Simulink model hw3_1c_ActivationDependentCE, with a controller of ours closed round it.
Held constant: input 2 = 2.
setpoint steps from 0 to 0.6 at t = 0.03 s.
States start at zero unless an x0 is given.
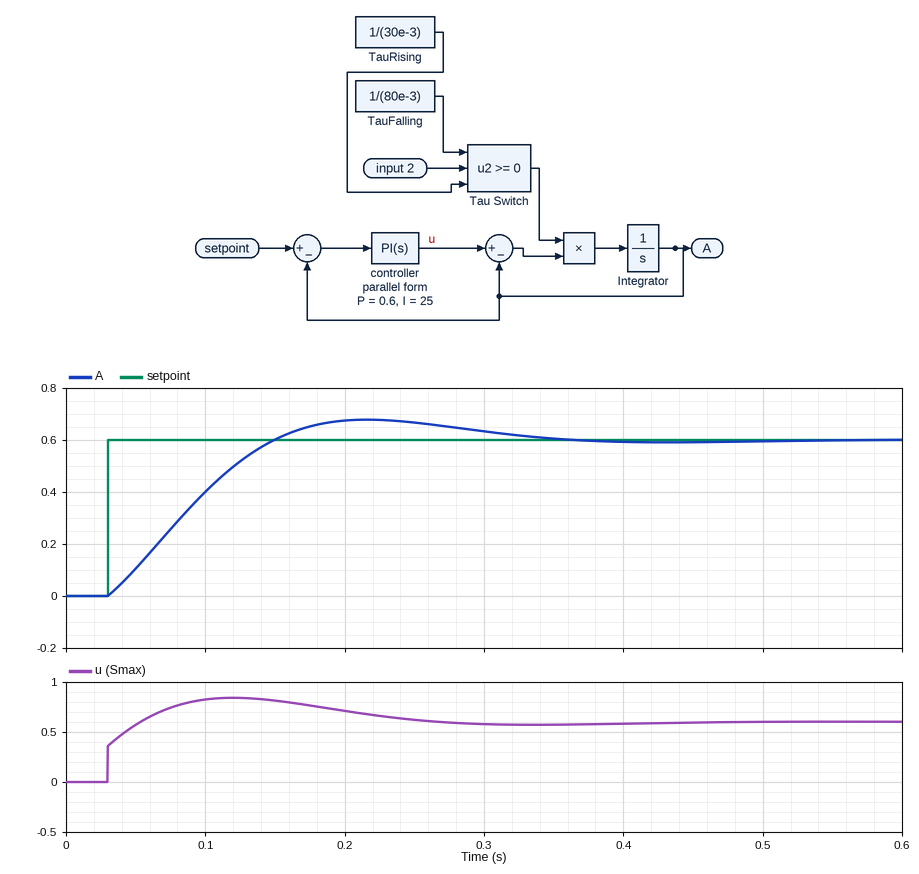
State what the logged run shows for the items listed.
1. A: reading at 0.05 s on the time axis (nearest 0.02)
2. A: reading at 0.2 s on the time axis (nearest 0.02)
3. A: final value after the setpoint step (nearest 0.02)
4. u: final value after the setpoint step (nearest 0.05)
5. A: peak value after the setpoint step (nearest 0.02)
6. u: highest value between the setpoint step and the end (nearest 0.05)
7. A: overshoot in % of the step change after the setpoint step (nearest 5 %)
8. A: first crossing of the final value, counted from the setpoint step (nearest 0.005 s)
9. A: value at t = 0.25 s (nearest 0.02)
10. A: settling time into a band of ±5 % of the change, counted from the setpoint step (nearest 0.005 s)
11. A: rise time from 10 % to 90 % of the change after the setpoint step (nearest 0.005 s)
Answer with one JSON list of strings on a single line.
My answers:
["0.10", "0.68", "0.60", "0.60", "0.68", "0.85", "15 %", "0.120 s", "0.66", "0.275 s", "0.090 s"]
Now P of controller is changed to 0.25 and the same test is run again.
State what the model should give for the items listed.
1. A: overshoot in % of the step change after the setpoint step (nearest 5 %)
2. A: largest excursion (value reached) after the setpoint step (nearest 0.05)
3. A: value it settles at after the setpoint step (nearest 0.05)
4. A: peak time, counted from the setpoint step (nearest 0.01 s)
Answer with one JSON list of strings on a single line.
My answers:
["20 %", "0.75", "0.60", "0.19 s"]
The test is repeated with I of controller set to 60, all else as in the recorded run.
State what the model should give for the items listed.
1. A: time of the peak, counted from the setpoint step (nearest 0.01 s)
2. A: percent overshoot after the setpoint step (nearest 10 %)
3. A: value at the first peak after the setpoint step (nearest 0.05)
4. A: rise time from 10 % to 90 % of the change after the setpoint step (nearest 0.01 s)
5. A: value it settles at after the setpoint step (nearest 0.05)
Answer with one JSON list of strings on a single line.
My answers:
["0.11 s", "30 %", "0.80", "0.05 s", "0.60"]
